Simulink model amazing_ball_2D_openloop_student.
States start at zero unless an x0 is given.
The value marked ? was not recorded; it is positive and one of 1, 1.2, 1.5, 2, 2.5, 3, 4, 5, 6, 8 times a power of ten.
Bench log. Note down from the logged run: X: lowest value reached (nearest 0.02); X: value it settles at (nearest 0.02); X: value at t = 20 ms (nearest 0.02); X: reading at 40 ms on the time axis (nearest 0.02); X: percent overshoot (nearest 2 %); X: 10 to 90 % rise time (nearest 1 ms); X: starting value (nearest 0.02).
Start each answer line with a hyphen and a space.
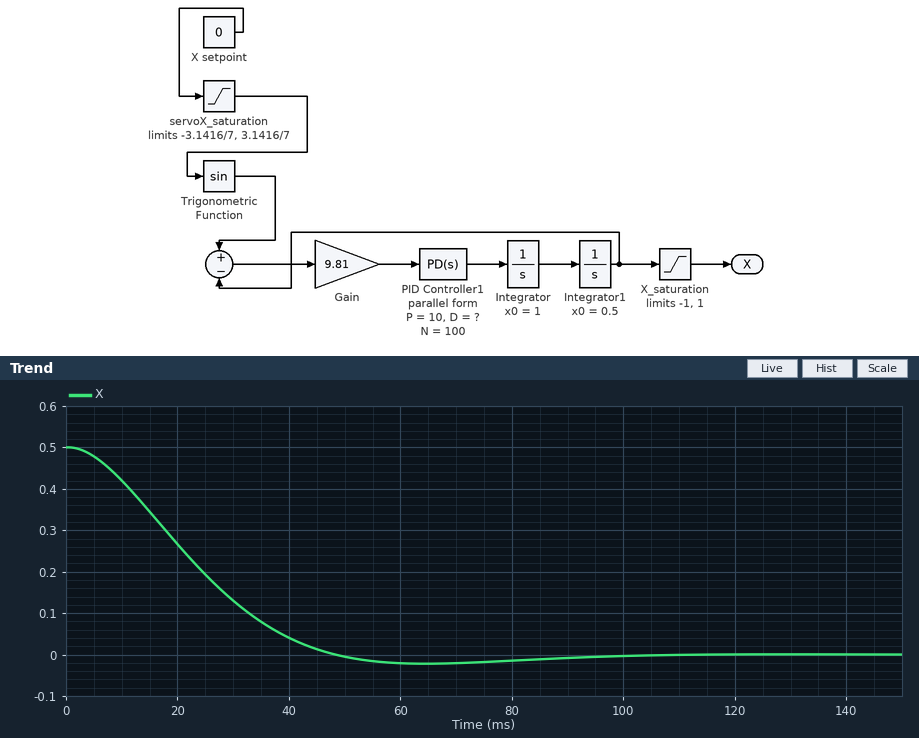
- -0.02
- 0.00
- 0.26
- 0.04
- 4 %
- 31 ms
- 0.50
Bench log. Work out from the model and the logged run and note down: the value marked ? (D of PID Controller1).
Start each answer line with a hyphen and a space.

- 5
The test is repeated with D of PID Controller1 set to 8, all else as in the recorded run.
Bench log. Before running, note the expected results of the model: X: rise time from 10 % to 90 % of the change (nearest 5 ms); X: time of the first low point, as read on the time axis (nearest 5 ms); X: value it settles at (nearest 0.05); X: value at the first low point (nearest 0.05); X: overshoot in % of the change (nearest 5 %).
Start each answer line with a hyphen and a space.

- 20 ms
- 45 ms
- 0.00
- -0.05
- 10 %
